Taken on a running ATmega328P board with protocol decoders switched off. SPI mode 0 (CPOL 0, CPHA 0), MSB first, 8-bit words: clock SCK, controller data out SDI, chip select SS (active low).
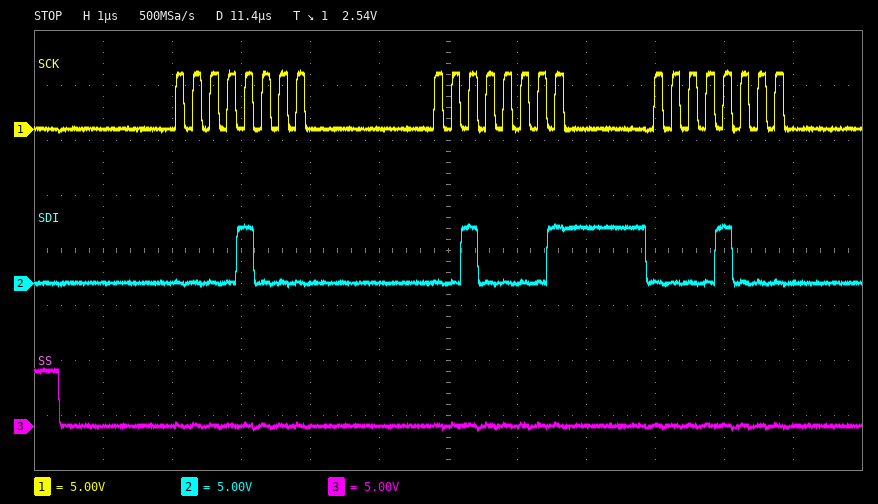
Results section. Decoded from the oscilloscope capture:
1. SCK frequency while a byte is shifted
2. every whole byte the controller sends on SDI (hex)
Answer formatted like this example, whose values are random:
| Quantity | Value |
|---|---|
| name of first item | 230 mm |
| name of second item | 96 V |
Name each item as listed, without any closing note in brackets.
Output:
| Quantity | Value |
|---|---|
| SCK frequency while a byte is shifted | 4 MHz |
| every whole byte the controller sends on SDI | 08 21 08 |
